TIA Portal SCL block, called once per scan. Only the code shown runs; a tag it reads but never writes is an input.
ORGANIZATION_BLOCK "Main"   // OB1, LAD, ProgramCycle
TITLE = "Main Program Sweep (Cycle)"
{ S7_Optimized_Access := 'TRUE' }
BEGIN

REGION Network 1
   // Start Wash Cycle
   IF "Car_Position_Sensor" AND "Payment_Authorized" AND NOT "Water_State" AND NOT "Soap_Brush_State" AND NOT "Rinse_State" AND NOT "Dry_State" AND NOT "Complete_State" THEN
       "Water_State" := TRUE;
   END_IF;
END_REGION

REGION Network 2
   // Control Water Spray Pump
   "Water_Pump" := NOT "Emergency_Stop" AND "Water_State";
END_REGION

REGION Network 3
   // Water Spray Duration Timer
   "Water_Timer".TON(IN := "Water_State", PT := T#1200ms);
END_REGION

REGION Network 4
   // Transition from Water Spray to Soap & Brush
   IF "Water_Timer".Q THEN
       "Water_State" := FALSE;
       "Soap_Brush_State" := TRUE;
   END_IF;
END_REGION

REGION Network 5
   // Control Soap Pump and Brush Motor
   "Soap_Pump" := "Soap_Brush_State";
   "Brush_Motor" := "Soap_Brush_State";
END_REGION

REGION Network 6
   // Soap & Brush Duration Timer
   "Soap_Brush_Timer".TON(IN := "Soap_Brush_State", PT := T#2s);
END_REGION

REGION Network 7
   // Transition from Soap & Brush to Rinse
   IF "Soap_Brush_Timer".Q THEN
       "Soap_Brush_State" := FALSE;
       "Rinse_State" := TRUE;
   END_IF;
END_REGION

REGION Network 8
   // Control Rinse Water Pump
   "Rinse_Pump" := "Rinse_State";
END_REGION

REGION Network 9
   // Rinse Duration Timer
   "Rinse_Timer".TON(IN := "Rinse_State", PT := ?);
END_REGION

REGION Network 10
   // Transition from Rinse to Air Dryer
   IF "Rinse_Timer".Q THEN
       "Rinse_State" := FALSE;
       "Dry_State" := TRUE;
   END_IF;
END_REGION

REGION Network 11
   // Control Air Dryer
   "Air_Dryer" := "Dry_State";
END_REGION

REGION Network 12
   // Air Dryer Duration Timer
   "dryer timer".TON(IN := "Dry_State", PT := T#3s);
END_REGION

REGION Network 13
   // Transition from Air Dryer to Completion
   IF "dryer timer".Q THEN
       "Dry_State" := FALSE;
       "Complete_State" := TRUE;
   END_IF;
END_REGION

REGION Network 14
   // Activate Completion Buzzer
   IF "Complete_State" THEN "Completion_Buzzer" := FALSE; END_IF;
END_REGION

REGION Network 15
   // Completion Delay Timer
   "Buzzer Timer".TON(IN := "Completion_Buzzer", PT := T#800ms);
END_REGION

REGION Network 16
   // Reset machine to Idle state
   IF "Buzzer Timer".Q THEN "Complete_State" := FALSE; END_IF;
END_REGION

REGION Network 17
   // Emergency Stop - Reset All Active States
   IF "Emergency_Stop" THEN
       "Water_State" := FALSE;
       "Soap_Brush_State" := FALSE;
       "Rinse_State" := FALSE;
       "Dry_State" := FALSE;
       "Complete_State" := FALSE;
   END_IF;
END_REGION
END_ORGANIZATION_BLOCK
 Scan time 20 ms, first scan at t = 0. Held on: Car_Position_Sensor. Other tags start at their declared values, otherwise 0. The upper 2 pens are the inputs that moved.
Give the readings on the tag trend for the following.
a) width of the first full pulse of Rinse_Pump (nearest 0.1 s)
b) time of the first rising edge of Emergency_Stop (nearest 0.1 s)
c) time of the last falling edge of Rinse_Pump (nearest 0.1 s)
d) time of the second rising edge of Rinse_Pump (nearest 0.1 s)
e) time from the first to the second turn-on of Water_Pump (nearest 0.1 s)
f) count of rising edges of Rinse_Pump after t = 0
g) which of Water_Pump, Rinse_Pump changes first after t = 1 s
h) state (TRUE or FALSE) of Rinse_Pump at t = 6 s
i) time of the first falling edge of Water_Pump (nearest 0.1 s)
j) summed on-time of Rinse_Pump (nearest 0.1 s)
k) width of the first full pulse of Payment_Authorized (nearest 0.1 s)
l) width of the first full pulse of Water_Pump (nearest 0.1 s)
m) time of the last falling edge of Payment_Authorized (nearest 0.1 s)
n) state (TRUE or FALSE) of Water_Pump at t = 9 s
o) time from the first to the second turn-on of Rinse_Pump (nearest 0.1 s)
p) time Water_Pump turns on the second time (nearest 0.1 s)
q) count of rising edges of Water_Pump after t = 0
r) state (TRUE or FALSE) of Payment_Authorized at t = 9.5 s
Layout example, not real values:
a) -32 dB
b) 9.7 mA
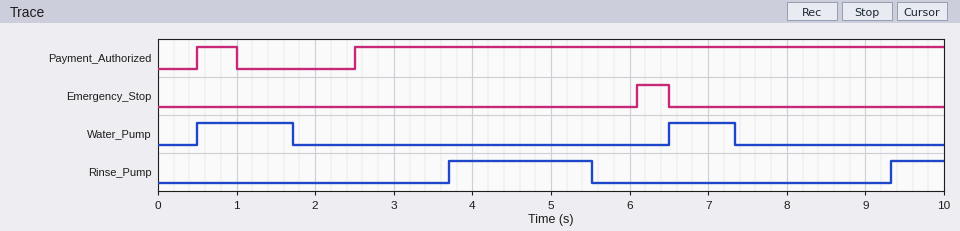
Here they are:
a) 1.8 s
b) 6.1 s
c) 5.5 s
d) 9.3 s
e) 6.0 s
f) 2
g) Water_Pump
h) FALSE
i) 1.7 s
j) 2.5 s
k) 0.5 s
l) 1.2 s
m) 1.0 s
n) FALSE
o) 5.6 s
p) 6.5 s
q) 2
r) TRUE
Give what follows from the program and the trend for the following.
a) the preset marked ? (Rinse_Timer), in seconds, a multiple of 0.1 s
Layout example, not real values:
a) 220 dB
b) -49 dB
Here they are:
a) 1.8 s
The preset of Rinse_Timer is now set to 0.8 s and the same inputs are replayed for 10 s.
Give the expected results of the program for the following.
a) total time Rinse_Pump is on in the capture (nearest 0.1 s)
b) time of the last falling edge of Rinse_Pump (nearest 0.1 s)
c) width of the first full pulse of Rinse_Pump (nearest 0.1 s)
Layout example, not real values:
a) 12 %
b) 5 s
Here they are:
a) 1.5 s
b) 4.5 s
c) 0.8 s
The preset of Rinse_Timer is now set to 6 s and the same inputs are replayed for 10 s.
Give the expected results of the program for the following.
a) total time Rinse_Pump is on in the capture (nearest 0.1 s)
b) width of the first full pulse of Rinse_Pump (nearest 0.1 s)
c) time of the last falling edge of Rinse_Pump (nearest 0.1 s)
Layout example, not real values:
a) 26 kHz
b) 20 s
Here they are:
a) 3.1 s
b) 2.4 s
c) 6.1 s
